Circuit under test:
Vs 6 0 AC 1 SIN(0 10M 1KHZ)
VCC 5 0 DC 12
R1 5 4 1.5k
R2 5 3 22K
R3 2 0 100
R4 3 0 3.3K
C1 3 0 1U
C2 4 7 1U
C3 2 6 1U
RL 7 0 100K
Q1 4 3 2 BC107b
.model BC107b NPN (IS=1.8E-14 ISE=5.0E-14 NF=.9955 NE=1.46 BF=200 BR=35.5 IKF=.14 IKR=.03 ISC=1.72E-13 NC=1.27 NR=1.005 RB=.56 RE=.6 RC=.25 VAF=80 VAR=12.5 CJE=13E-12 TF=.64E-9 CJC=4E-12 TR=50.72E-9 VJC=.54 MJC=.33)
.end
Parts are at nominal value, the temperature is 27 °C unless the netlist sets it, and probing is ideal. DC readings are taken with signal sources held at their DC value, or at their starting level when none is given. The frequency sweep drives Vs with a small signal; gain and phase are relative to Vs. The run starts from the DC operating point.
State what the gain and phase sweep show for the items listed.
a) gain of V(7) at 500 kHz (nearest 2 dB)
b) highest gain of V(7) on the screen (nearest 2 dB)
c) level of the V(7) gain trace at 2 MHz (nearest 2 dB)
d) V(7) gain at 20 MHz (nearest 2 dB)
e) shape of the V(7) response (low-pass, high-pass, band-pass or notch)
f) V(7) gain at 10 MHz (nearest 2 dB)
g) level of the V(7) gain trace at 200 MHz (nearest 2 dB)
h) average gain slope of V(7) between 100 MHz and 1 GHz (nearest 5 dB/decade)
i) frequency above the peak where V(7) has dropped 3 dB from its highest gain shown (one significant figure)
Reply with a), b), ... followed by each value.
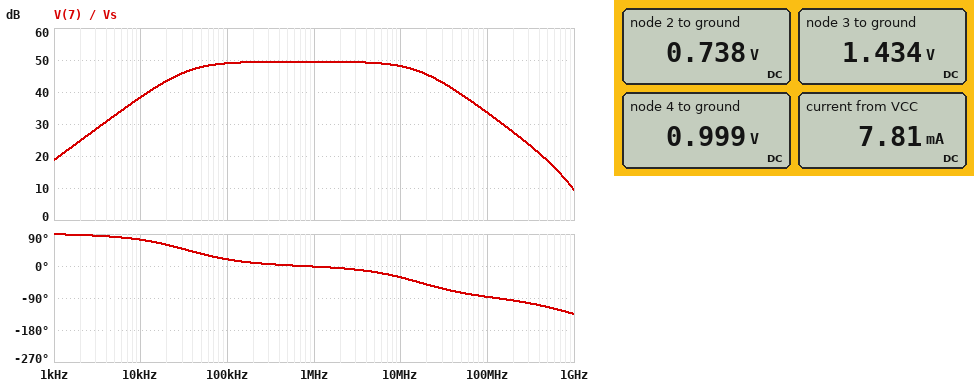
a) 50 dB
b) 50 dB
c) 50 dB
d) 46 dB
e) band-pass
f) 48 dB
g) 28 dB
h) -25 dB/decade
i) 20 MHz
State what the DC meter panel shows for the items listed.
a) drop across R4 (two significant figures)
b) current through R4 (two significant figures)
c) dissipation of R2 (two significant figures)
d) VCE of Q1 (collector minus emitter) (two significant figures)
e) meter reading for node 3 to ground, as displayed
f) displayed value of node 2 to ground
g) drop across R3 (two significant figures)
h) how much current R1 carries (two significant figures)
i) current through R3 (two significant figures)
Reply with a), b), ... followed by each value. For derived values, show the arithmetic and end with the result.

a) 1.434 V = 1.4 V
b) (1.434 V) / 3.3 kΩ = 430 µA
c) (12 V - 1.434 V)^2 / 22 kΩ = 5.1 mW
d) 999 mV - 738 mV = 260 mV
e) 1.434 V
f) 0.738 V
g) 738 mV = 740 mV
h) (12 V - 999 mV) / 1.5 kΩ = 7.3 mA
i) (738 mV) / 100 Ω = 7.4 mA
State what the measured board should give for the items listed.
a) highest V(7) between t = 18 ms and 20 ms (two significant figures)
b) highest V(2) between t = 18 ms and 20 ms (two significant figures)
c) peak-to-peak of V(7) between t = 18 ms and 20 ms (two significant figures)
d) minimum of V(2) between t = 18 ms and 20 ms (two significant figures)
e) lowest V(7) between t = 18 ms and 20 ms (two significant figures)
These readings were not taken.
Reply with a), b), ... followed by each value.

a) 93 mV
b) 740 mV
c) 170 mV
d) 740 mV
e) -78 mV
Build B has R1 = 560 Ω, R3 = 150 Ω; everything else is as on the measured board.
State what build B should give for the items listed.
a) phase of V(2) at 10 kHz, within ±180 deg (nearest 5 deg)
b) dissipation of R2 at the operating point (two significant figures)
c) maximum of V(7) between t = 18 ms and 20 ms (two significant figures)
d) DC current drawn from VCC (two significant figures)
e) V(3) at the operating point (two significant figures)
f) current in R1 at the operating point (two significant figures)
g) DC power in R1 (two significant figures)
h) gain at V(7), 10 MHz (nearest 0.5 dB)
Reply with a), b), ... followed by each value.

a) 70 deg
b) 5.0 mW
c) 33 mV
d) 5.8 mA
e) 1.5 V
f) 5.3 mA
g) 16 mW
h) 39.5 dB
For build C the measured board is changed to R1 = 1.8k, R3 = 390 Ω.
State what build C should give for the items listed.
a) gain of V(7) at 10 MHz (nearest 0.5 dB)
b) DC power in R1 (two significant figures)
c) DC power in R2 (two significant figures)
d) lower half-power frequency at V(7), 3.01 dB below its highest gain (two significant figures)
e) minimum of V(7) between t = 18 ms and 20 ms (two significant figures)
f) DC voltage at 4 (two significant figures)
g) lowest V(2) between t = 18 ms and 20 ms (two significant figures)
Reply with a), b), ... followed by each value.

a) 42.5 dB
b) 8.9 mW
c) 5.0 mW
d) 13 kHz
e) -110 mV
f) 8.0 V
g) 870 mV
